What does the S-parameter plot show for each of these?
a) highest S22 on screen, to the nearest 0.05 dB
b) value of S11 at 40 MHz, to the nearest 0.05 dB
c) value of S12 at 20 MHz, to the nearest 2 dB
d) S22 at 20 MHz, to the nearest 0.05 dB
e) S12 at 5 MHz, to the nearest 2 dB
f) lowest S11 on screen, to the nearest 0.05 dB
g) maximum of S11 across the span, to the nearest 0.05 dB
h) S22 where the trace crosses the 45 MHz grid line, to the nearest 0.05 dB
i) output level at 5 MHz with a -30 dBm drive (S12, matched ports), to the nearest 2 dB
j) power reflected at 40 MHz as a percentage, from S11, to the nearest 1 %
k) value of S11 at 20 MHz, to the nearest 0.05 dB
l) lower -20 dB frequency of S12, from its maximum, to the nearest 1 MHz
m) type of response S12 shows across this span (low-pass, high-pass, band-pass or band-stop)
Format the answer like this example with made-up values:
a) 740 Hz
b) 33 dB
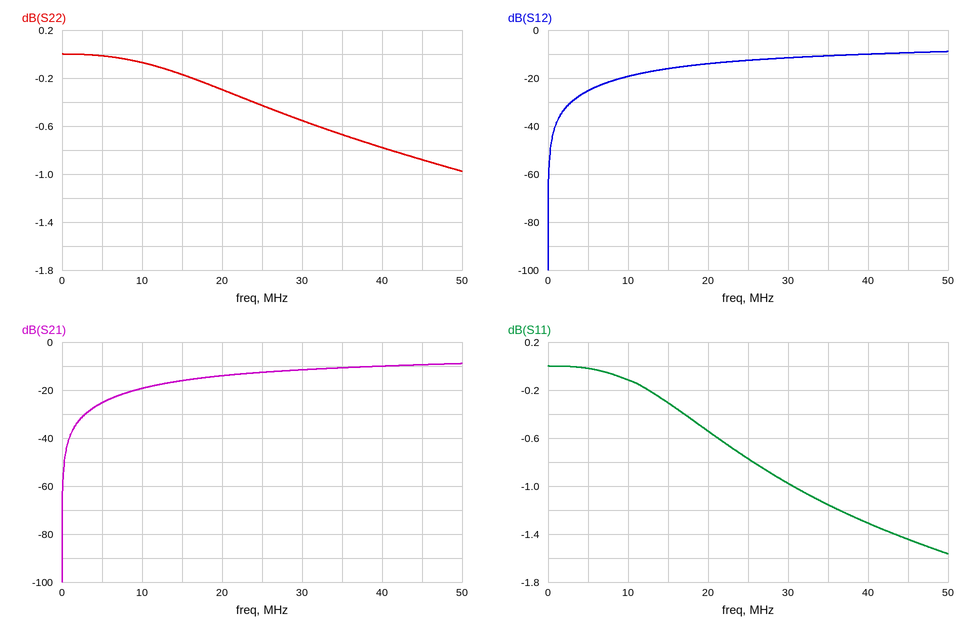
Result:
a) 0.00 dB
b) -1.30 dB
c) -14 dB
d) -0.30 dB
e) -26 dB
f) -1.55 dB
g) 0.00 dB
h) -0.90 dB
i) -56 dBm
j) 74 %
k) -0.55 dB
l) 3 MHz
m) high-pass
